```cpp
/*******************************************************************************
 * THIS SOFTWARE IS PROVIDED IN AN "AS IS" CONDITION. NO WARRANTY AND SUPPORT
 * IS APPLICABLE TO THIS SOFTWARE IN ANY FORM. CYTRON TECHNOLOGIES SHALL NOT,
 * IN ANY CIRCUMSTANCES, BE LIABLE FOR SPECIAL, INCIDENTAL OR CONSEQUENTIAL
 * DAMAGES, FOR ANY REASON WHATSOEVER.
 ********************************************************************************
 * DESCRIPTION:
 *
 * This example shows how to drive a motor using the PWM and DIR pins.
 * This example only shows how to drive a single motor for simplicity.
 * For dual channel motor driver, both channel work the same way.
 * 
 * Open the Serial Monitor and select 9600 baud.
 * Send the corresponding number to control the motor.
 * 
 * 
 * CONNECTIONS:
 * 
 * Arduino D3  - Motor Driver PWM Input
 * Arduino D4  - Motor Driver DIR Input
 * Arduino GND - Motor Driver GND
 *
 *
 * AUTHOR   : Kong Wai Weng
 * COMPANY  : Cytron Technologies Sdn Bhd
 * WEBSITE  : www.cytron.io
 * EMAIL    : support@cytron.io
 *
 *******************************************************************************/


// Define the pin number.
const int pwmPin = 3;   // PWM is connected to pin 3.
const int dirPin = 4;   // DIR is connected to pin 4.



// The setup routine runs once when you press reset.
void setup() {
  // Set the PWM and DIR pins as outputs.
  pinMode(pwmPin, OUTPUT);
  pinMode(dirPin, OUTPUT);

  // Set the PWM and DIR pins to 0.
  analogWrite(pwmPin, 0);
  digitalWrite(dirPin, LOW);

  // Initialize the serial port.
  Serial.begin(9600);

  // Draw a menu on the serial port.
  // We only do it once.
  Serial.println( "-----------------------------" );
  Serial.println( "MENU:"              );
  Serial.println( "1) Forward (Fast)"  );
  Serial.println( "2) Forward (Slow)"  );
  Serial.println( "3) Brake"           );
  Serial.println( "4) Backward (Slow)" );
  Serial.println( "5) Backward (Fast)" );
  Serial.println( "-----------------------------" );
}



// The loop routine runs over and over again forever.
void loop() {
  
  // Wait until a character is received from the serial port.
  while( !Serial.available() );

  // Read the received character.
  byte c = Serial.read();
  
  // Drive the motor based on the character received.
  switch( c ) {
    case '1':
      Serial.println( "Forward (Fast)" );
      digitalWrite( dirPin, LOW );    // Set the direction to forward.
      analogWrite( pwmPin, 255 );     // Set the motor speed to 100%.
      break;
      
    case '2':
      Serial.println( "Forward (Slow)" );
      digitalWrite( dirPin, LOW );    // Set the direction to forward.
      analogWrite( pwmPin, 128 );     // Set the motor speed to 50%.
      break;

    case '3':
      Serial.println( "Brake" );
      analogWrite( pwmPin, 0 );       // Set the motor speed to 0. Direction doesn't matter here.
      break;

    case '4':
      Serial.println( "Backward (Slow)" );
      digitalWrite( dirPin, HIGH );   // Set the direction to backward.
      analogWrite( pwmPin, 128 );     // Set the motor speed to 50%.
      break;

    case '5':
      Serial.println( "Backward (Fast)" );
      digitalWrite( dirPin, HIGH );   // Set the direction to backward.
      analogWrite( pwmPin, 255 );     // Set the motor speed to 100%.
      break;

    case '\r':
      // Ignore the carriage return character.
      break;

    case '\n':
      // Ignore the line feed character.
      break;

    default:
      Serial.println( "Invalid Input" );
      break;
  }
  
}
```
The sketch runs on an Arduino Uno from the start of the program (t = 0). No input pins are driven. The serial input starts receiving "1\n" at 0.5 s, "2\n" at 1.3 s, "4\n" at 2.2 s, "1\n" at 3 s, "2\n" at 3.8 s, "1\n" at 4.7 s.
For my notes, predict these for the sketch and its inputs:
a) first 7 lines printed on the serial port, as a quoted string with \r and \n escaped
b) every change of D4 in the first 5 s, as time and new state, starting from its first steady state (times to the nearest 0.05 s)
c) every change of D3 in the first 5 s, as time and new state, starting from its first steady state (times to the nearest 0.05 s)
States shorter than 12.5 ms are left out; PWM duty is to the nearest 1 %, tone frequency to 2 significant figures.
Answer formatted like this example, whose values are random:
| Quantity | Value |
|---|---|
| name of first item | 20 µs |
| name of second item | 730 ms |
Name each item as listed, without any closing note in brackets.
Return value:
| Quantity | Value |
|---|---|
| first 7 lines printed on the serial port, as a quoted string with \r and \n escaped | "-----------------------------\r\nMENU:\r\n1) Forward (Fast)\r\n2) Forward (Slow)\r\n3) Brake\r\n4) Backward (Slow)\r\n5) Backward (Fast)\r\n" |
| every change of D4 in the first 5 s, as time and new state, starting from its first steady state | 0 s low; 2.2 s high; 3 s low |
| every change of D3 in the first 5 s, as time and new state, starting from its first steady state | 0 s low; 0.5 s high; 1.3 s PWM 50 %; 3 s high; 3.8 s PWM 50 %; 4.7 s high |
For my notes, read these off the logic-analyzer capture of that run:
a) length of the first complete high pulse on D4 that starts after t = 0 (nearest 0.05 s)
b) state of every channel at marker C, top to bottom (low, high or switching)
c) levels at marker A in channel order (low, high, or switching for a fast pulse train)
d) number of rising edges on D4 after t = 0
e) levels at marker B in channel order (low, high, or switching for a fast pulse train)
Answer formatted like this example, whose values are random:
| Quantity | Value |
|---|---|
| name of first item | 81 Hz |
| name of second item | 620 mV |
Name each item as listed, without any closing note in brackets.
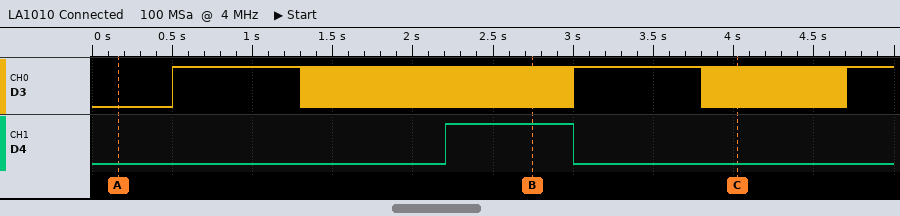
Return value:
| Quantity | Value |
|---|---|
| length of the first complete high pulse on D4 that starts after t = 0 | 0.80 s |
| state of every channel at marker C, top to bottom | D3 switching, D4 low |
| levels at marker A in channel order | D3 low, D4 low |
| number of rising edges on D4 after t = 0 | 1 |
| levels at marker B in channel order | D3 switching, D4 high |
